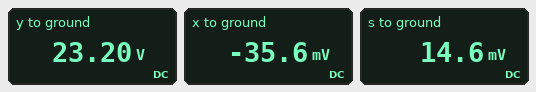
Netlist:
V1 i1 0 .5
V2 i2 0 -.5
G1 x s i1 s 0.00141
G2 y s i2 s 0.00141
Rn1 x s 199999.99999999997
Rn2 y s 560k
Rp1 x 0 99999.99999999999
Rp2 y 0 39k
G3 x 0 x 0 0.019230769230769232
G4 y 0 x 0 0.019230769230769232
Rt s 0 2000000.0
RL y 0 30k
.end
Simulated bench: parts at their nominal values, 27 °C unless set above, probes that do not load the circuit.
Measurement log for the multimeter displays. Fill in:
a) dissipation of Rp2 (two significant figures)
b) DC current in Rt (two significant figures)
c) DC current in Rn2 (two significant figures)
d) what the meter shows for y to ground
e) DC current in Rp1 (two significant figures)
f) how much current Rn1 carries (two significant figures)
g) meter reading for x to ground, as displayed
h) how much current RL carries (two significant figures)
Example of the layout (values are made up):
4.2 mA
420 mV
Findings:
14 mW
7.3 nA
41 µA
23.20 V
360 nA
250 nA
-35.6 mV
770 µA
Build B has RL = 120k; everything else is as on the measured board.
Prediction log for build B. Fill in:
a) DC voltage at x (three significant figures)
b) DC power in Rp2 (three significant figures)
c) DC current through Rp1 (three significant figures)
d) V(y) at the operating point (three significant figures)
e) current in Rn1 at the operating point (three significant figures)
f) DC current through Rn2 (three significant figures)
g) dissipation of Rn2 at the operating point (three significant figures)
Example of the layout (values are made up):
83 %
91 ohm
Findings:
-34.8 mV
39.8 mW
348 nA
39.4 V
298 nA
70.3 µA
2.77 mW
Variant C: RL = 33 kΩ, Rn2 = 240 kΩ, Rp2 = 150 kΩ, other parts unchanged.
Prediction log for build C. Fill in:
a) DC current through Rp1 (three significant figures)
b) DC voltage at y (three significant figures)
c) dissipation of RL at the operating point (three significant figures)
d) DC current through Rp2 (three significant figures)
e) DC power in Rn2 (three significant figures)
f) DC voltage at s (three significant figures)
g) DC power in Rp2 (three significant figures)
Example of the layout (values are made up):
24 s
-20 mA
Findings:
329 nA
34.3 V
35.6 mW
228 µA
4.88 mW
50.4 mV
7.83 mW
